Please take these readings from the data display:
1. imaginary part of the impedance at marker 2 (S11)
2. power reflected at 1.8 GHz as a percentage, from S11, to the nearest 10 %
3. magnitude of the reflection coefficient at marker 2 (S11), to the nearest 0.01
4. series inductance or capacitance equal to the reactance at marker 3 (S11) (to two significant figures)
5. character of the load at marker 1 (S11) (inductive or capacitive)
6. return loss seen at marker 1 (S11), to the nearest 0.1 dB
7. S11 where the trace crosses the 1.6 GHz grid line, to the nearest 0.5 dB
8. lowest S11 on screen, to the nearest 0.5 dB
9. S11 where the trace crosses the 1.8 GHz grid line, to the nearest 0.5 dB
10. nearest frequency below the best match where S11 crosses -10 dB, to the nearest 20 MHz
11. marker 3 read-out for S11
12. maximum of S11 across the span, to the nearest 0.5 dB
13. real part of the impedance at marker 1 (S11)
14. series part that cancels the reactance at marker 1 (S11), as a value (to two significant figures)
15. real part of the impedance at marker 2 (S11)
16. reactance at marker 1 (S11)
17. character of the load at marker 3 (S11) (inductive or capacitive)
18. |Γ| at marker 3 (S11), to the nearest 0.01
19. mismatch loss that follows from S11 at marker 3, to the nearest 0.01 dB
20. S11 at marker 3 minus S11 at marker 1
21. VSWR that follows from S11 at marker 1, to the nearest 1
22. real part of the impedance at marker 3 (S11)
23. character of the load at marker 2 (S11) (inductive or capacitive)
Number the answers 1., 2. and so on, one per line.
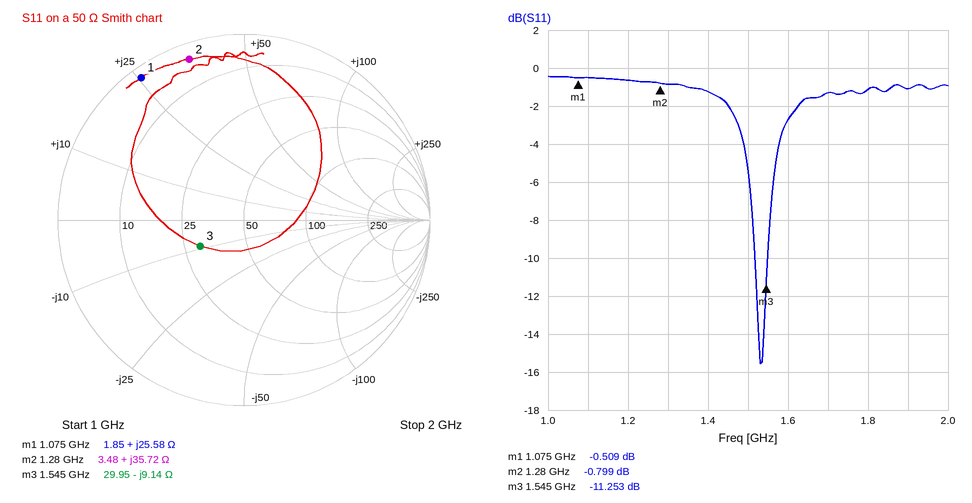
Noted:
1. +35.72 Ω
2. 80 %
3. 0.91
4. 11 pF
5. inductive
6. 0.5 dB
7. -2.5 dB
8. -15.5 dB
9. -1.0 dB
10. 1.52 GHz
11. -11.253 dB
12. -0.5 dB
13. 1.85 Ω
14. 5.8 pF
15. 3.48 Ω
16. +25.58 Ω
17. capacitive
18. 0.27
19. 0.34 dB
20. -10.744 dB
21. 34
22. 29.95 Ω
23. inductive
